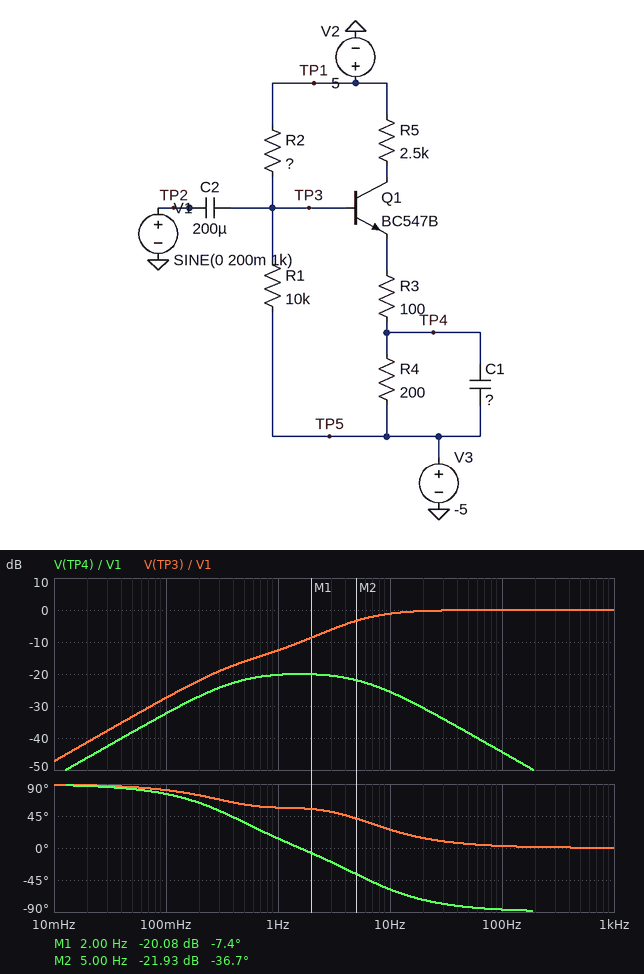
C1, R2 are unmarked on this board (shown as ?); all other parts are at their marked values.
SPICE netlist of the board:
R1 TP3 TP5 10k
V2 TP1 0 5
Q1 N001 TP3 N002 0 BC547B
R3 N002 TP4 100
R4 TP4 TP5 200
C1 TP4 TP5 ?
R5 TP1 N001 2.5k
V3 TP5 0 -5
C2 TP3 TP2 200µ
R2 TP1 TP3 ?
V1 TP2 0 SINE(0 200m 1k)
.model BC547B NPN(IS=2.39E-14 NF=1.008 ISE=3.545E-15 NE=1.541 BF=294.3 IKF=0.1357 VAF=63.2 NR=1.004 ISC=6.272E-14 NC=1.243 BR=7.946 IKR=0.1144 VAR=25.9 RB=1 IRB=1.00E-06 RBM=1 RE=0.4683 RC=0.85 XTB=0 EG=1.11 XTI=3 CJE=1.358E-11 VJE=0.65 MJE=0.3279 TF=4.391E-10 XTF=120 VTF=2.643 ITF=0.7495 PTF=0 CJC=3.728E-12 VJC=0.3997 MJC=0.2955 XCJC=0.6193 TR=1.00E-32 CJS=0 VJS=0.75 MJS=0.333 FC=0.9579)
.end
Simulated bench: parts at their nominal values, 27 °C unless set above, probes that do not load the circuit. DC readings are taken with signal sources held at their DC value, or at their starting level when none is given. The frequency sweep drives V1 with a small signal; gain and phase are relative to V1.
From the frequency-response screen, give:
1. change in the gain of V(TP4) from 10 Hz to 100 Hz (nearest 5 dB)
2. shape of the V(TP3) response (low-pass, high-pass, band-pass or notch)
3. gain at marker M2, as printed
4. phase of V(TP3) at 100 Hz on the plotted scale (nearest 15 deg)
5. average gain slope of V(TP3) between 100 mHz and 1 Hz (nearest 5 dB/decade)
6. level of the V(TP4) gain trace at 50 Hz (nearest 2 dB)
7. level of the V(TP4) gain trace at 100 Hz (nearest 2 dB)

-20 dB
high-pass
-21.93 dB
0 deg
15 dB/decade
-38 dB
-44 dB
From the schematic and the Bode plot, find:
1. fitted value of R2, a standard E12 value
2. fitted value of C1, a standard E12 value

33 kΩ
1.8 mF
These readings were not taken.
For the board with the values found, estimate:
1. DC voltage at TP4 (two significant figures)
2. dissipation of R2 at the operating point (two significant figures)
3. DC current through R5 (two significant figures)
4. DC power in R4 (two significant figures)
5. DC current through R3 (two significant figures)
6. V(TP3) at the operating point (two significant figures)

-4.3 V
2.1 mW
3.5 mA
2.6 mW
3.6 mA
-3.2 V
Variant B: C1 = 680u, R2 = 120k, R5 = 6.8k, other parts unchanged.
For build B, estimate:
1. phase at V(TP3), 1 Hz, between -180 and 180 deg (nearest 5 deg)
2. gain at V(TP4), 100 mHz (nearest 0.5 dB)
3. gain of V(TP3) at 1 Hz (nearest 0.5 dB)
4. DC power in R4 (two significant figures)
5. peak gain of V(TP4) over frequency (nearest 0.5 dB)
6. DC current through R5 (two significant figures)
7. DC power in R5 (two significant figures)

5 deg
-8.0 dB
0 dB
43 µW
-5.5 dB
460 µA
1.5 mW
